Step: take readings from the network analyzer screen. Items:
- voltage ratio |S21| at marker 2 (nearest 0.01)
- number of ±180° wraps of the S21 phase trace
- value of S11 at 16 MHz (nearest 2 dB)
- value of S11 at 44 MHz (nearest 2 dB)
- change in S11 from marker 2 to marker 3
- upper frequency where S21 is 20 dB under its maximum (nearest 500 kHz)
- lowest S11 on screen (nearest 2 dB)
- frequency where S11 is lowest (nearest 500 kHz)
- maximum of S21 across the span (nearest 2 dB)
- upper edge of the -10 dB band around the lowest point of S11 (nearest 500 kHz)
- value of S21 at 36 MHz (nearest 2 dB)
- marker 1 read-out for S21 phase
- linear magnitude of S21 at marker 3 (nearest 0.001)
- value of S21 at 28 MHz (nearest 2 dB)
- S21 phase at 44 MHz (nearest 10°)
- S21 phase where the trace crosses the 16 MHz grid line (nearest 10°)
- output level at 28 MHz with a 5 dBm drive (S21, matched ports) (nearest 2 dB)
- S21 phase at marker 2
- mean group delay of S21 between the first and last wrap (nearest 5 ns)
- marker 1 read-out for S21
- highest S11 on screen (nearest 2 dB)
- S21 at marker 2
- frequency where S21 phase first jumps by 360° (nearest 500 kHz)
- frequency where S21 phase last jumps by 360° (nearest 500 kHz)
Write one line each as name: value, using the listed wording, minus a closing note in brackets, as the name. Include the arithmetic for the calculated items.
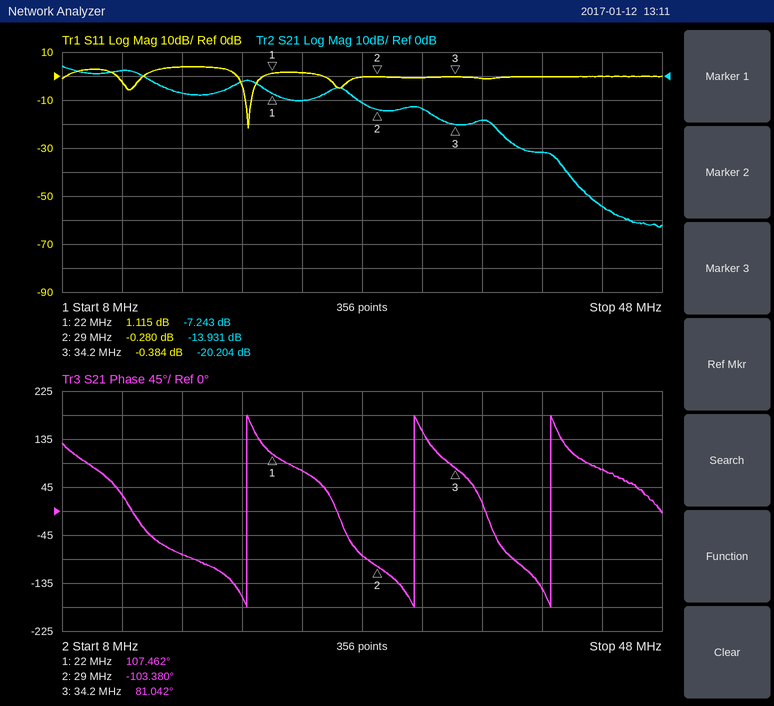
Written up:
voltage ratio |S21| at marker 2: 10^(-13.931/20) ≈ 0.20
number of ±180° wraps of the S21 phase trace: 3
value of S11 at 16 MHz: 4 dB
value of S11 at 44 MHz: 0 dB
change in S11 from marker 2 to marker 3: -0.384 − (-0.28) = -0.104 dB
upper frequency where S21 is 20 dB under its maximum: 32.5 MHz
lowest S11 on screen: -22 dB
frequency where S11 is lowest: 20.5 MHz
maximum of S21 across the span: 4 dB
upper edge of the -10 dB band around the lowest point of S11: 20.5 MHz
value of S21 at 36 MHz: -18 dB
marker 1 read-out for S21 phase: 107.462°
linear magnitude of S21 at marker 3: 10^(-20.204/20) ≈ 0.098
value of S21 at 28 MHz: -12 dB
S21 phase at 44 MHz: 80°
S21 phase where the trace crosses the 16 MHz grid line: -80°
output level at 28 MHz with a 5 dBm drive (S21, matched ports): 5 dBm + (-12 dB) = -6 dBm
S21 phase at marker 2: -103.380°
mean group delay of S21 between the first and last wrap: 2 cycles / (40.5 MHz − 20.5 MHz) ≈ 100 ns
marker 1 read-out for S21: -7.243 dB
highest S11 on screen: 4 dB
S21 at marker 2: -13.931 dB
frequency where S21 phase first jumps by 360°: 20.5 MHz
frequency where S21 phase last jumps by 360°: 40.5 MHz
